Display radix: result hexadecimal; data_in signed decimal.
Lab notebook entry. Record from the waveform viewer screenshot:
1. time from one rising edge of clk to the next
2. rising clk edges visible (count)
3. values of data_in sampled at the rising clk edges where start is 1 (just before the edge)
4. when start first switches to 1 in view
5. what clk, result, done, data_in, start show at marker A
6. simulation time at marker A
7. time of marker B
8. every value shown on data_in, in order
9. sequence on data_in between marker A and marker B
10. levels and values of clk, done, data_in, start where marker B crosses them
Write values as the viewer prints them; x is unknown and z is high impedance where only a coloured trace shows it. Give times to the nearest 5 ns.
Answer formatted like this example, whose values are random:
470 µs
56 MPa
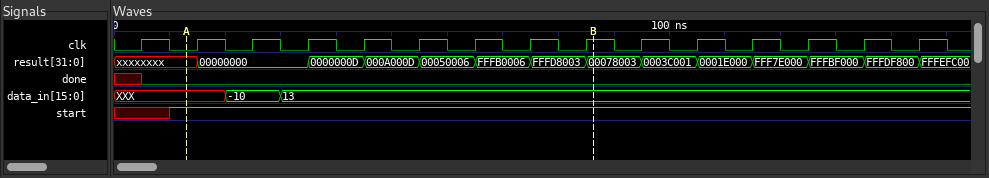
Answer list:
10 ns
15
XXX, -10, 13, 13, 13, 13, 13, 13, 13, 13, 13, 13, 13, 13
10 ns
clk=0, result=xxxxxxxx, done=0, data_in=XXX, start=1
15 ns
85 ns
XXX, -10, 13
XXX, -10, 13
clk=1, done=0, data_in=13, start=1
